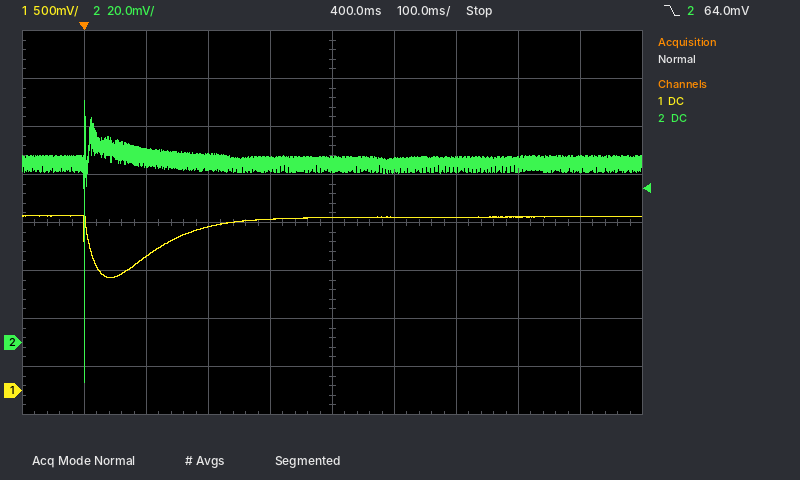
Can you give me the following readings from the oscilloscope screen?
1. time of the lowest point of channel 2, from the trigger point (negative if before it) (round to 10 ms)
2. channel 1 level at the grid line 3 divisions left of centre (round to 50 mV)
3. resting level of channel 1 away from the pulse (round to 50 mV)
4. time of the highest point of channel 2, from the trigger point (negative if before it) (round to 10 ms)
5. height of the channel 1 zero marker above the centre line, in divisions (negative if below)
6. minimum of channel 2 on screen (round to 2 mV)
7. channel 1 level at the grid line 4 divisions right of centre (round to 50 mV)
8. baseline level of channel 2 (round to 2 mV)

0 ms
1.40 V
1.80 V
0 ms
-3.5 div
-16 mV
1.80 V
74 mV
